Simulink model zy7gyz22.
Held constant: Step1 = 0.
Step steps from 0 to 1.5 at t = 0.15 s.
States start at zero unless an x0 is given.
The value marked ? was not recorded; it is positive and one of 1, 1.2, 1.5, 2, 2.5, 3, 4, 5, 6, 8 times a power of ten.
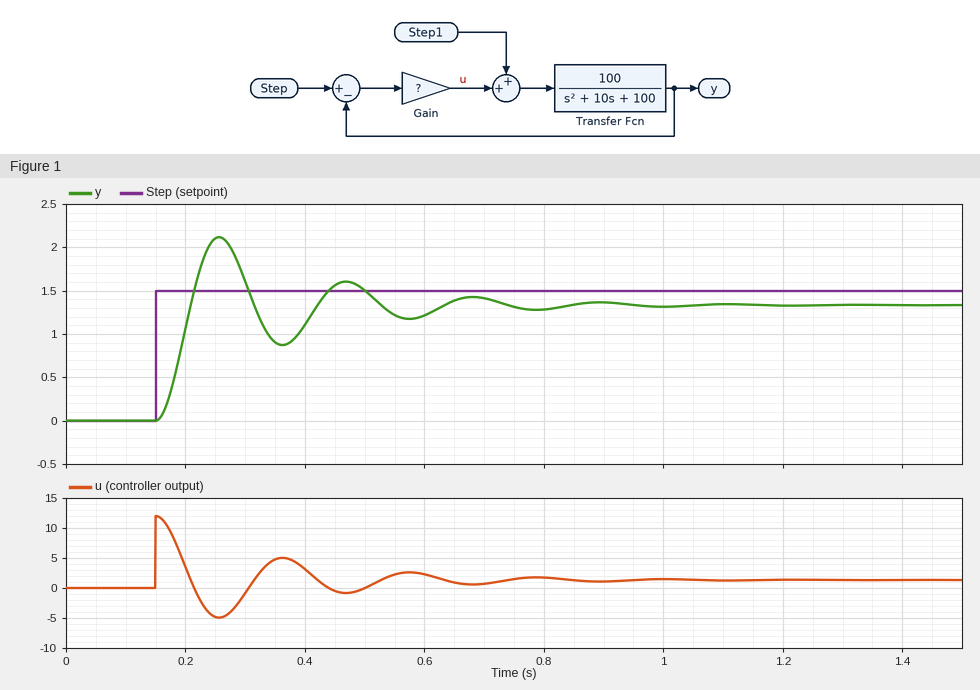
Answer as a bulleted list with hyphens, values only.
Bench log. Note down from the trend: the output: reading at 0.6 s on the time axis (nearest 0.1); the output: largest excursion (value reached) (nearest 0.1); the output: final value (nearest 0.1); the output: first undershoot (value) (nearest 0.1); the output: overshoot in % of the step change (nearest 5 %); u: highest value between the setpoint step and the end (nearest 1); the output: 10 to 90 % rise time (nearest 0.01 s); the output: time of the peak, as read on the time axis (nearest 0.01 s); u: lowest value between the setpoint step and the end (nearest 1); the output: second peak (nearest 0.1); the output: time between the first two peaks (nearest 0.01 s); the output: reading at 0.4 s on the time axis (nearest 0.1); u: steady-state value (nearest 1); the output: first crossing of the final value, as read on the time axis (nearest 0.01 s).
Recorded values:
- 1.2
- 2.1
- 1.3
- 0.9
- 60 %
- 12
- 0.04 s
- 0.26 s
- -5
- 1.6
- 0.21 s
- 1.1
- 1
- 0.21 s
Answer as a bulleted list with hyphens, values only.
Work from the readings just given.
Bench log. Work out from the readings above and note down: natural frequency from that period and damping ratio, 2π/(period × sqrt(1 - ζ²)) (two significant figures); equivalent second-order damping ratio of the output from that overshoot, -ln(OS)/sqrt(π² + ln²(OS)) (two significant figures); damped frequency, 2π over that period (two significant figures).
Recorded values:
- 30 rad/s
- 0.16
- 30 rad/s
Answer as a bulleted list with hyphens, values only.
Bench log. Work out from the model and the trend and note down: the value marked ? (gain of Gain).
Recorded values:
- 8
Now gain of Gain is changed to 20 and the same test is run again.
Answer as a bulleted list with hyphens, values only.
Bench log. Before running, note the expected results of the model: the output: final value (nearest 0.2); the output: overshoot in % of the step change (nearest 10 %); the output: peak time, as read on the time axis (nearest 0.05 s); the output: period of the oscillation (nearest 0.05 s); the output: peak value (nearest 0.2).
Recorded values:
- 1.4
- 70 %
- 0.20 s
- 0.15 s
- 2.4
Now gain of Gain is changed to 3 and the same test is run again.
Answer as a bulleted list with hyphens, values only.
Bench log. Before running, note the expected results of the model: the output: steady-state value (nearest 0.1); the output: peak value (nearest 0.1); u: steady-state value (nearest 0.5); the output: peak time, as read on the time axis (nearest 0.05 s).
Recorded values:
- 1.1
- 1.6
- 1.0
- 0.30 s
